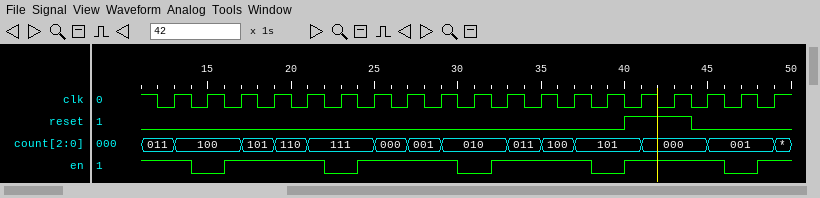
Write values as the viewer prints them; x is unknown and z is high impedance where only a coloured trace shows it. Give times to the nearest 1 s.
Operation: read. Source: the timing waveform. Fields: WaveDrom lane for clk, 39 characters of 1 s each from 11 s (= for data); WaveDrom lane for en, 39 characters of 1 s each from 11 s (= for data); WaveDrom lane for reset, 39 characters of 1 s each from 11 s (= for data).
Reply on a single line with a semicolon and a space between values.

{name: 'clk', wave: '101010101010101010101010101010101010101'}; {name: 'en', wave: '1..0.1.....0.1.....0.1.....0.1.....0.1.'}; {name: 'reset', wave: '0............................1...0.....'}
